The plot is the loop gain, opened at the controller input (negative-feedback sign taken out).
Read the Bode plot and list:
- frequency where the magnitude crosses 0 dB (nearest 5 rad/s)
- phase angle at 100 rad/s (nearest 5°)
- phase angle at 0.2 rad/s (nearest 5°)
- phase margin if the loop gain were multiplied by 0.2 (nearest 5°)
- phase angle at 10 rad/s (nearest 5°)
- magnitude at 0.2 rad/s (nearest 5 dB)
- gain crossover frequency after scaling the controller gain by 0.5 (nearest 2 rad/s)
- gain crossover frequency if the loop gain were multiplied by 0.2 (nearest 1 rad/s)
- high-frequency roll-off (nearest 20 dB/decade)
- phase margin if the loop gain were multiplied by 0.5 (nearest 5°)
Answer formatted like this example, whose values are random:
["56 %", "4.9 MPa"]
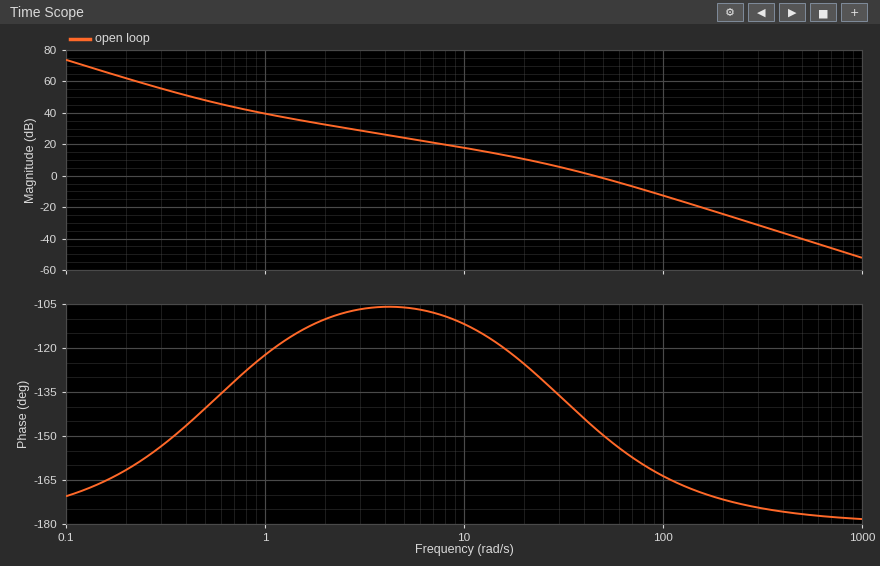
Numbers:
["45 rad/s", "-165°", "-160°", "60°", "-110°", "60 dB", "30 rad/s", "15 rad/s", "-40 dB/decade", "45°"]
